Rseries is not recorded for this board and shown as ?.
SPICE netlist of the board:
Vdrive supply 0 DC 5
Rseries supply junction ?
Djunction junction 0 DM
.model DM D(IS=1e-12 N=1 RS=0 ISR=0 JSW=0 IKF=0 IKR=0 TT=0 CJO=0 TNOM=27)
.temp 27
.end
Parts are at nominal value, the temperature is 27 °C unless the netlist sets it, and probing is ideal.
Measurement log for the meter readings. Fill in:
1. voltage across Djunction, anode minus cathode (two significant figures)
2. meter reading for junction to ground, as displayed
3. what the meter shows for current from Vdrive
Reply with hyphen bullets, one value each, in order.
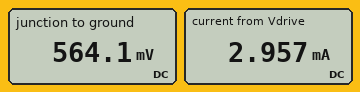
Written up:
- 560 mV
- 564.1 mV
- 2.957 mA
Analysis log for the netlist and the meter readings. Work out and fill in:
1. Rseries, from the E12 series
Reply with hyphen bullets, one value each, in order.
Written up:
- 1.5 kΩ
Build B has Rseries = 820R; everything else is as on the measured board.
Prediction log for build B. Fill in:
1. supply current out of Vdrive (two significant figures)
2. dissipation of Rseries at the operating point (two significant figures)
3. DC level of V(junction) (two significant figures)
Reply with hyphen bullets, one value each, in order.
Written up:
- 5.4 mA
- 24 mW
- 580 mV
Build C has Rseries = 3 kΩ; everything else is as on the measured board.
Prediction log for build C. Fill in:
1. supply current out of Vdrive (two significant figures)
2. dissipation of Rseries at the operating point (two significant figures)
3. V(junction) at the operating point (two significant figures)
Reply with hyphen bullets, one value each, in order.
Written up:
- 1.5 mA
- 6.6 mW
- 550 mV
